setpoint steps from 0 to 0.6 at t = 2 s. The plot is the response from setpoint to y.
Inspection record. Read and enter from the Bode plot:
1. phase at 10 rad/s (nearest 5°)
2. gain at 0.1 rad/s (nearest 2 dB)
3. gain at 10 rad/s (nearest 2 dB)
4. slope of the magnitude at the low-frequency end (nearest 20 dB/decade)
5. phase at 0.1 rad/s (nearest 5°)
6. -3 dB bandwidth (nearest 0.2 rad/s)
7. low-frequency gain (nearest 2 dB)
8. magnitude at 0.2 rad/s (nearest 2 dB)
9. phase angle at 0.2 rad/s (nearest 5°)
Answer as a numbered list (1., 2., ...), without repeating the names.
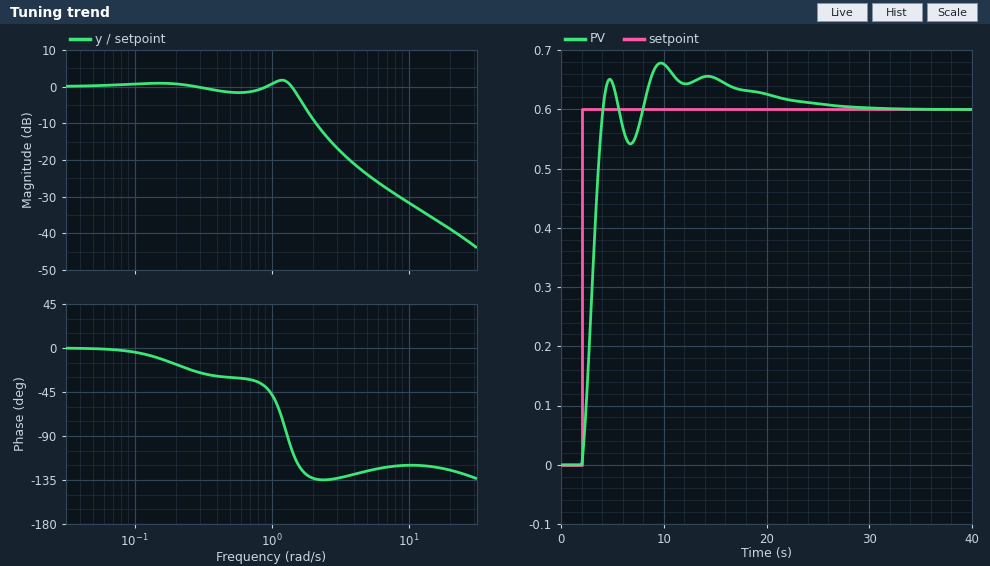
1. -120°
2. 0 dB
3. -32 dB
4. 0 dB/decade
5. -5°
6. 1.6 rad/s
7. 0 dB
8. 0 dB
9. -15°
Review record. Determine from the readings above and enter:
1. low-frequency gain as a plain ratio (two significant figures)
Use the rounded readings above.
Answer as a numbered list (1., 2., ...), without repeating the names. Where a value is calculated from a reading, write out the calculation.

1. 10^(0 / 20) = 1.0
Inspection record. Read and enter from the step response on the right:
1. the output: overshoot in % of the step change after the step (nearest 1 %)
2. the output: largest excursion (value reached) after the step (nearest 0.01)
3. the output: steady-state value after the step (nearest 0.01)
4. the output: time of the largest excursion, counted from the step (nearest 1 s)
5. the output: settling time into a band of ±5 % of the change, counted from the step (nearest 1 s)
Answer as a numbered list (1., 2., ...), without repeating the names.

1. 13 %
2. 0.68
3. 0.60
4. 8 s
5. 17 s
